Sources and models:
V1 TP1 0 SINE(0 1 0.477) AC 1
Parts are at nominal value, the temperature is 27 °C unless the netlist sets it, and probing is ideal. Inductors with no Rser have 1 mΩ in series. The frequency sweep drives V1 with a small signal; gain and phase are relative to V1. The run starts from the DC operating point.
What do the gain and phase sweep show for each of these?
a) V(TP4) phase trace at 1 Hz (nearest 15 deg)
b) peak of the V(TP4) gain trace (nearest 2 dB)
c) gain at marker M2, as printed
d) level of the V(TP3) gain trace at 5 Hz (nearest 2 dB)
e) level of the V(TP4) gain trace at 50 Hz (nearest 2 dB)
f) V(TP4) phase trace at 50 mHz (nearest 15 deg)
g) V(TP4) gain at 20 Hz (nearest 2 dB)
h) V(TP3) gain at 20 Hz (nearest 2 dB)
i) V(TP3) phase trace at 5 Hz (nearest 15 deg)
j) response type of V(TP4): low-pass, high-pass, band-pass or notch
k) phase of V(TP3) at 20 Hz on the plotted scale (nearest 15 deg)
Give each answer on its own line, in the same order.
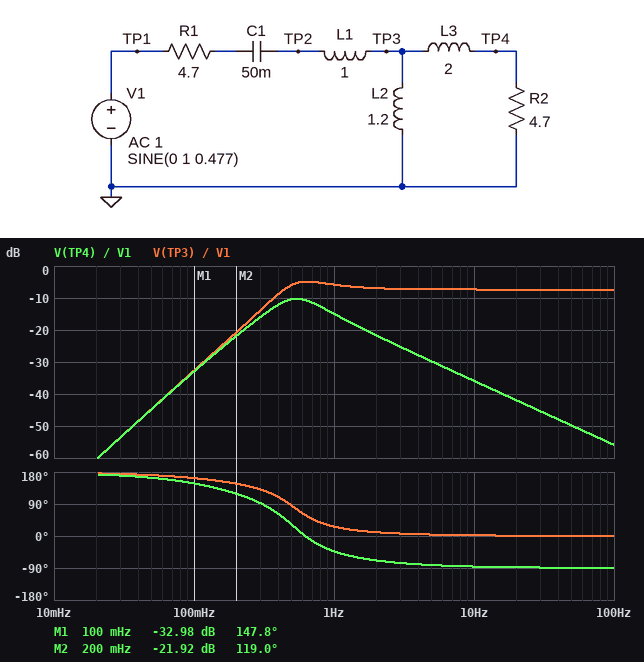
-45 deg
-10 dB
-21.92 dB
-8 dB
-50 dB
165 deg
-42 dB
-8 dB
0 deg
band-pass
0 deg
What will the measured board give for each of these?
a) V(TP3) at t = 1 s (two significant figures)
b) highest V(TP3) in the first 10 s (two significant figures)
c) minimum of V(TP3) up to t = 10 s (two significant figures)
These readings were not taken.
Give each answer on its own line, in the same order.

-350 mV
480 mV
-480 mV
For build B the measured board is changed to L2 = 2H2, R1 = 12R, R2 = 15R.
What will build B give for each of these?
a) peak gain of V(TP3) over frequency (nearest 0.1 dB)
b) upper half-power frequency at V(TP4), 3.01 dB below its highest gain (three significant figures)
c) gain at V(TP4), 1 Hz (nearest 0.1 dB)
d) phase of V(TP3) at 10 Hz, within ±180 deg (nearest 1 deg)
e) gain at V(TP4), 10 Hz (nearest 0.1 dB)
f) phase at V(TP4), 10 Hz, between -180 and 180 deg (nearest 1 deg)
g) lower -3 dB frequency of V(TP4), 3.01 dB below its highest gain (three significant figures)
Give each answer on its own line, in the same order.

-5.8 dB
1.80 Hz
-8.9 dB
4 deg
-24.4 dB
-80 deg
308 mHz
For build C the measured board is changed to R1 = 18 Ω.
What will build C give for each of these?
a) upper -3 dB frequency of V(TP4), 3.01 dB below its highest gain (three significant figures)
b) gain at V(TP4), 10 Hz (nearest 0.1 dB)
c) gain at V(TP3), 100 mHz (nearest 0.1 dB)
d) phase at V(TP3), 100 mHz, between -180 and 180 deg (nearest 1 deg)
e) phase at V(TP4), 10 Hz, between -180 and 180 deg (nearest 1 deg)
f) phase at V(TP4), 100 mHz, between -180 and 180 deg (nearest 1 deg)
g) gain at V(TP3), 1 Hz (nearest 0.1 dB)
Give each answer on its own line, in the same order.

2.03 Hz
-36.0 dB
-33.9 dB
141 deg
-79 deg
126 deg
-12.3 dB
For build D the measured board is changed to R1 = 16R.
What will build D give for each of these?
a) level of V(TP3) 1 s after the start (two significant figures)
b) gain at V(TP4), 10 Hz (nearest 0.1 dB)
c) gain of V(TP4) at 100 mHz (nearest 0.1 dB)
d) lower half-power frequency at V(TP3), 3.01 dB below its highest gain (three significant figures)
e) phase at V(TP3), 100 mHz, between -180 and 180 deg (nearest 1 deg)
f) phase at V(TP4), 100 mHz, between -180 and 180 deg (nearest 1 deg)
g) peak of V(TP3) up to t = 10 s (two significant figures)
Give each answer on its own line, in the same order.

-140 mV
-36.0 dB
-33.9 dB
1.27 Hz
144 deg
129 deg
160 mV
